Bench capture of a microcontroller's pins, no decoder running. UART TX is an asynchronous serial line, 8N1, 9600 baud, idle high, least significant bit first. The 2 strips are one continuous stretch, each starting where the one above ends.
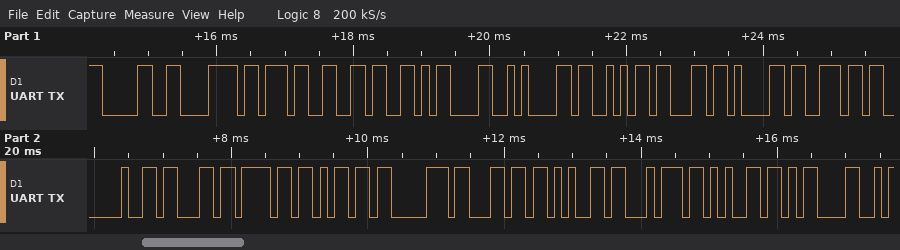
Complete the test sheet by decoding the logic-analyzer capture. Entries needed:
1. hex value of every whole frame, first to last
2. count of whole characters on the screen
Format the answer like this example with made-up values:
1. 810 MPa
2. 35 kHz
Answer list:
1. 30 78 37 36 0D 0A 53 63 61 6E 20 63 6F 6D 70 6C 65 74 65 0D
2. 20
